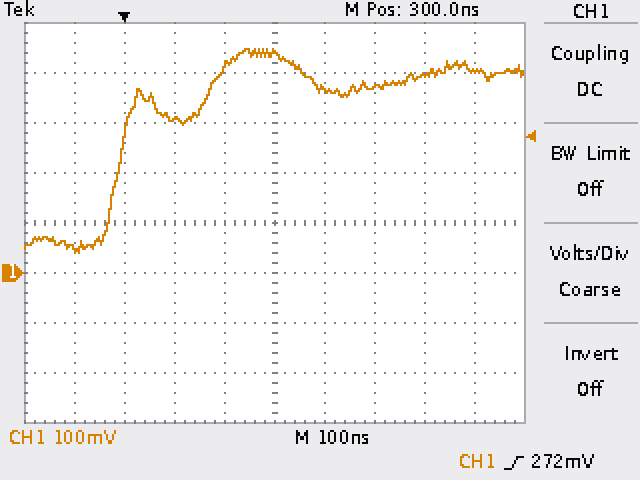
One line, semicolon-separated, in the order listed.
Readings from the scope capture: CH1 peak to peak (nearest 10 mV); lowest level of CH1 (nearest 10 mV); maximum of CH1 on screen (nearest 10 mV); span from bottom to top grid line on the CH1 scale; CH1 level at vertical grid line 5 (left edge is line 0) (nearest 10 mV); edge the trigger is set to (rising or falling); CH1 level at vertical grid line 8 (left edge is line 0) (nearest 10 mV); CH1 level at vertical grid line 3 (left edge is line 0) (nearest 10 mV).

410 mV; 40 mV; 450 mV; 800 mV; 440 mV; rising; 400 mV; 310 mV
